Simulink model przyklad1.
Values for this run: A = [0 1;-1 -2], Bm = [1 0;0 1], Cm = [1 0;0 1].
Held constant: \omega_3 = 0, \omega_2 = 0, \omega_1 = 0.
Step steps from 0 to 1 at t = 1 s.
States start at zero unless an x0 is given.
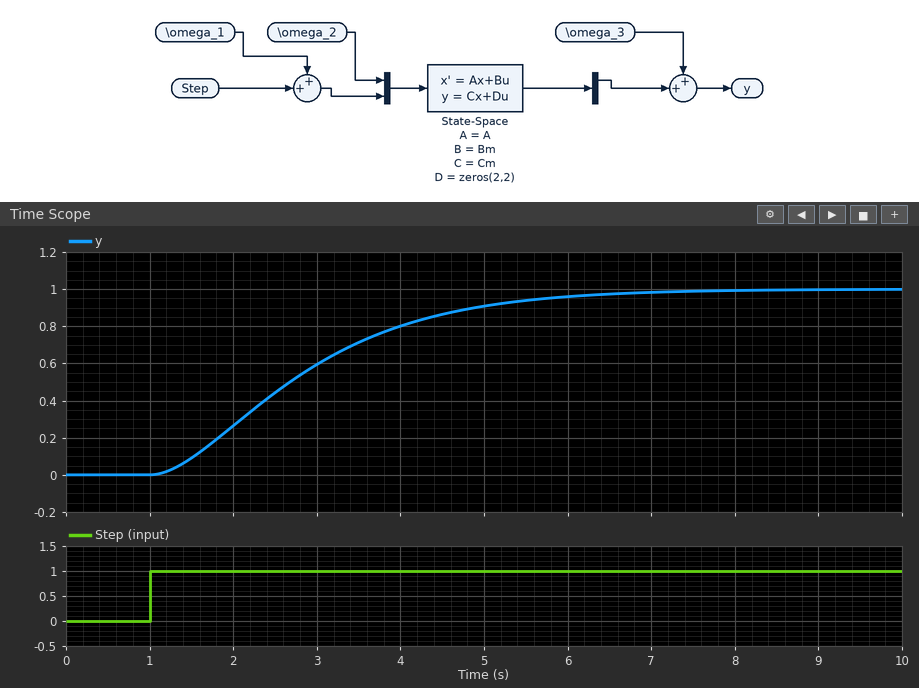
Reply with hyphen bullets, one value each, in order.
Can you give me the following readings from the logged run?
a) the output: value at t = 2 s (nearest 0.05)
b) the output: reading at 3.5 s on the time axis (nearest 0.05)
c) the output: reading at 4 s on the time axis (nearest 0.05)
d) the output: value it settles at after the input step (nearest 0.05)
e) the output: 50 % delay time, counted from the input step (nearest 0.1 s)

- 0.25
- 0.70
- 0.80
- 1.00
- 1.7 s
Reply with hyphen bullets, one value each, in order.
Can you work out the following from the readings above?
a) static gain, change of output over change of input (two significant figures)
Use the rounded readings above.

- 1.0
